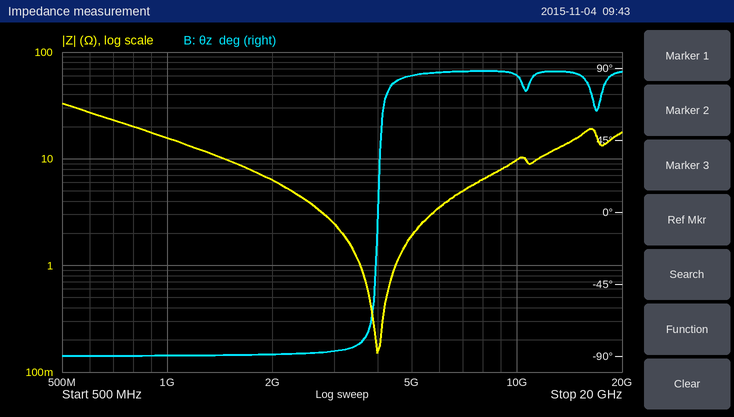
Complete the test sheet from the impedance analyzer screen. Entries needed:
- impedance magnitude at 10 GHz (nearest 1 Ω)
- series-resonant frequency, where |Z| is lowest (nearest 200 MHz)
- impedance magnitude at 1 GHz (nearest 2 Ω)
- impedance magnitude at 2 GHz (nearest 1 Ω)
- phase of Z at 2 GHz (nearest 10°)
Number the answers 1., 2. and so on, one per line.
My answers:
1. 10 Ω
2. 4.0 GHz
3. 16 Ω
4. 6 Ω
5. -90°
